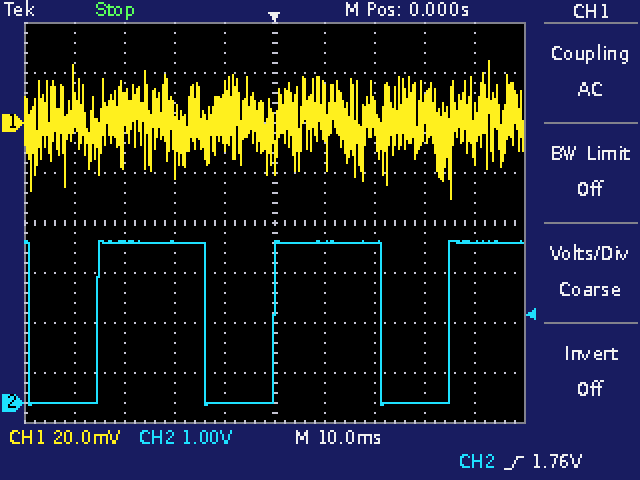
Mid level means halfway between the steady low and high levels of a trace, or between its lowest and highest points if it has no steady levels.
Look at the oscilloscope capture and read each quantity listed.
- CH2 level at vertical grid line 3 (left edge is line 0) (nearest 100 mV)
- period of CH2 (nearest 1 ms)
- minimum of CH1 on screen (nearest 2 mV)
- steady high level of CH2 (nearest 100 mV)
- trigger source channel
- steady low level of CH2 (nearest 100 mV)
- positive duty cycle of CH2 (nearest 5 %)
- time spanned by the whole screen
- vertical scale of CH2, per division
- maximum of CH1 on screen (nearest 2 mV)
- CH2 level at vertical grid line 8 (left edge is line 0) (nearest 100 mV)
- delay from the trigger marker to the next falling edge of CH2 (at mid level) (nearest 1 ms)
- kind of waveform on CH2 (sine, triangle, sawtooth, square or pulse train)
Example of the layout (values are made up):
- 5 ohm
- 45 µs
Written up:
- 3.2 V
- 35 ms
- -30 mV
- 3.2 V
- CH2
- 0.0 V
- 60 %
- 100 ms
- 1 V
- 24 mV
- 0.0 V
- 21 ms
- pulse train
